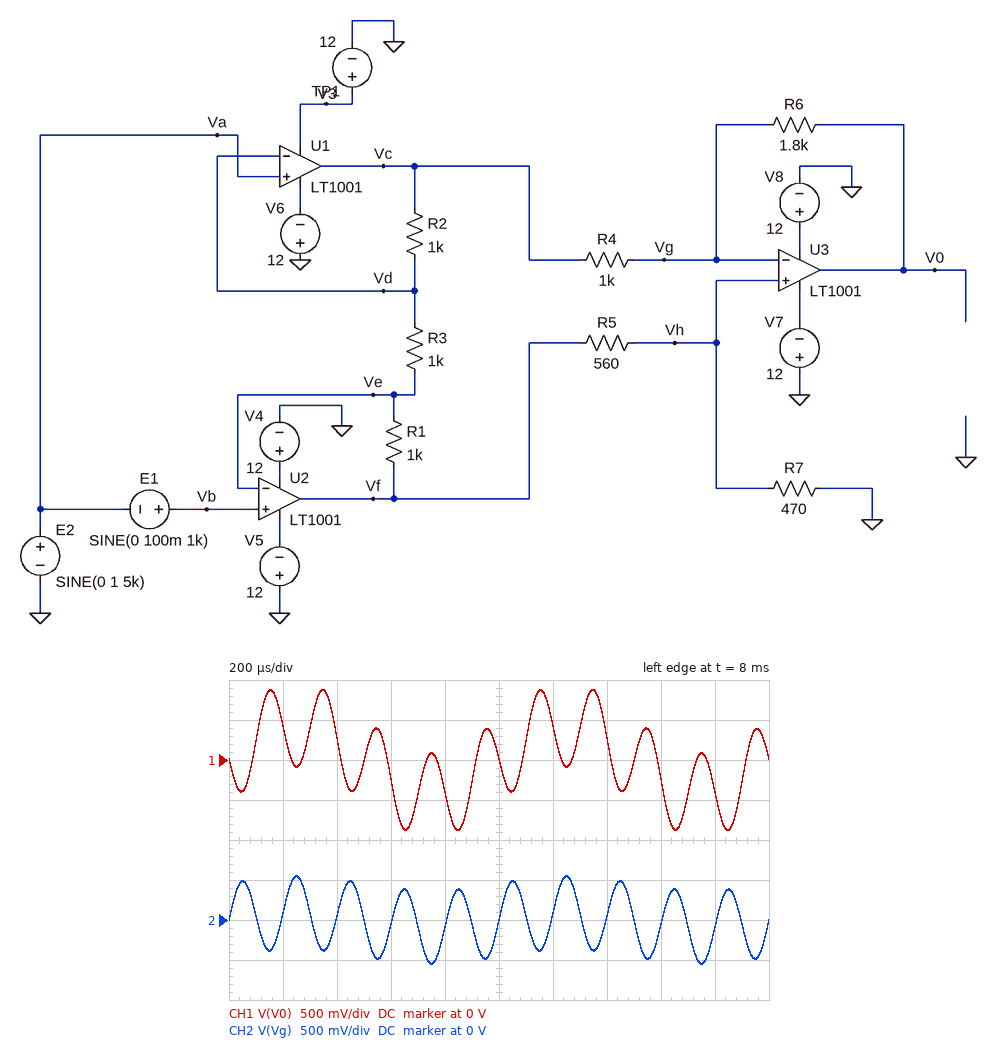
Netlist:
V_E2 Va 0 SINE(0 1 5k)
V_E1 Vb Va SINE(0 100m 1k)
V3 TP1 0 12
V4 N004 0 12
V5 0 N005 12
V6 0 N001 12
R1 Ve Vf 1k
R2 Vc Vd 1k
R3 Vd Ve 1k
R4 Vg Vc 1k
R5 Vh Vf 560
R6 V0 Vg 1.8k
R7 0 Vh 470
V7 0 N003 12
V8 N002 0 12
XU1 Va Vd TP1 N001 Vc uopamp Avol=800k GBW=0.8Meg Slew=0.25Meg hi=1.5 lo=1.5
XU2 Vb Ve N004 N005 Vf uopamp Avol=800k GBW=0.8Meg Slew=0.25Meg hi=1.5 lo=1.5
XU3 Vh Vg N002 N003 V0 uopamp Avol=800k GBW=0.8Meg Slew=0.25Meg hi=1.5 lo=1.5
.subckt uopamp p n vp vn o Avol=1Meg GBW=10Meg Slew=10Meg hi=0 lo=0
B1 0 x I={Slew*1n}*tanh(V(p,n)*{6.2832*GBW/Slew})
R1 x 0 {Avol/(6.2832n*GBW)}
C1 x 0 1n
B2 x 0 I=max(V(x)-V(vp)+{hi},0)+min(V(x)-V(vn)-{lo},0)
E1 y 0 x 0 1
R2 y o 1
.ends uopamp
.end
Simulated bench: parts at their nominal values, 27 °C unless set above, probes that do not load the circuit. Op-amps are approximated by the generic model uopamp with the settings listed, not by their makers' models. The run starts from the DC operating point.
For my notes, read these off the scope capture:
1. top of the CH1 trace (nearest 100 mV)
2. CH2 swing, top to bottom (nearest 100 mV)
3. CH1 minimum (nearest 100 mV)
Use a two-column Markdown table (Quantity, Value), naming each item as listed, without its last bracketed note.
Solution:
| Quantity | Value |
|---|---|
| top of the CH1 trace | 900 mV |
| CH2 swing, top to bottom | 1.1 V |
| CH1 minimum | -900 mV |
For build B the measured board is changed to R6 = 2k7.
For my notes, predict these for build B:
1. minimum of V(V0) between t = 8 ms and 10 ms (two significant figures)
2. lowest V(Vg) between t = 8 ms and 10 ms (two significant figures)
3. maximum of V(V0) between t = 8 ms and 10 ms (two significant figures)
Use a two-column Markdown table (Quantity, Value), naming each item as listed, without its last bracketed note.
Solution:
| Quantity | Value |
|---|---|
| minimum of V(V0) between t = 8 ms and 10 ms | -1.5 V |
| lowest V(Vg) between t = 8 ms and 10 ms | -550 mV |
| maximum of V(V0) between t = 8 ms and 10 ms | 1.5 V |
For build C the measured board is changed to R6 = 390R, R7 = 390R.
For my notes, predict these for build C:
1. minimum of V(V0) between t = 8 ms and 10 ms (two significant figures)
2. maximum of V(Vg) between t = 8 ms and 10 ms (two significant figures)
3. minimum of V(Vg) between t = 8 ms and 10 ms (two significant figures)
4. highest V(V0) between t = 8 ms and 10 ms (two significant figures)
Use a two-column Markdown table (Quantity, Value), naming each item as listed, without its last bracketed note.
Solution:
| Quantity | Value |
|---|---|
| minimum of V(V0) between t = 8 ms and 10 ms | -330 mV |
| maximum of V(Vg) between t = 8 ms and 10 ms | 490 mV |
| minimum of V(Vg) between t = 8 ms and 10 ms | -490 mV |
| highest V(V0) between t = 8 ms and 10 ms | 330 mV |
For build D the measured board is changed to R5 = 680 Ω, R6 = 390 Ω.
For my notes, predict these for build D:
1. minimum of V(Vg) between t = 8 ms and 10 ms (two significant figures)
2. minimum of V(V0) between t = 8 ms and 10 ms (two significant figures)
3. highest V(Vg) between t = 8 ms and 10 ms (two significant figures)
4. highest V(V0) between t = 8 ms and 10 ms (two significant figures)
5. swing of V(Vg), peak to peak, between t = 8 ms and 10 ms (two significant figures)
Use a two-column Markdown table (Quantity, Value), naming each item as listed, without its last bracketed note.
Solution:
| Quantity | Value |
|---|---|
| minimum of V(Vg) between t = 8 ms and 10 ms | -490 mV |
| minimum of V(V0) between t = 8 ms and 10 ms | -330 mV |
| highest V(Vg) between t = 8 ms and 10 ms | 490 mV |
| highest V(V0) between t = 8 ms and 10 ms | 330 mV |
| swing of V(Vg), peak to peak, between t = 8 ms and 10 ms | 980 mV |
